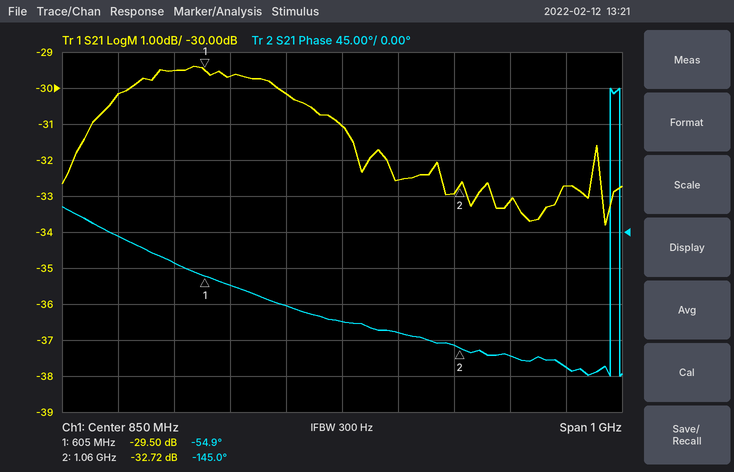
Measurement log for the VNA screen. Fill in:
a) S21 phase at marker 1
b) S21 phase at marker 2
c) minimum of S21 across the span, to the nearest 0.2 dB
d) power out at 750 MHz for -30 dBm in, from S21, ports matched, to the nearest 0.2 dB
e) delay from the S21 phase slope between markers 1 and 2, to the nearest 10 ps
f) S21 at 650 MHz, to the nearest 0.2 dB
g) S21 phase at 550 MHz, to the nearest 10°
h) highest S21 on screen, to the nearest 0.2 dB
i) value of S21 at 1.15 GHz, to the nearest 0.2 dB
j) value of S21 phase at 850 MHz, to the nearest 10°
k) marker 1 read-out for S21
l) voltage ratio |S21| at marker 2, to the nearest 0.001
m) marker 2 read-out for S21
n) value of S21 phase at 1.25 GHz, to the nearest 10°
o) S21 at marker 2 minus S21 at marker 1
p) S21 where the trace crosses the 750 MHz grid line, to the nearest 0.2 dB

-54.9°
-145.0°
-33.8 dB
-60.2 dBm
550 ps
-29.6 dB
-40°
-29.4 dB
-33.2 dB
-110°
-29.50 dB
0.023
-32.72 dB
-170°
-3.22 dB
-30.2 dB
